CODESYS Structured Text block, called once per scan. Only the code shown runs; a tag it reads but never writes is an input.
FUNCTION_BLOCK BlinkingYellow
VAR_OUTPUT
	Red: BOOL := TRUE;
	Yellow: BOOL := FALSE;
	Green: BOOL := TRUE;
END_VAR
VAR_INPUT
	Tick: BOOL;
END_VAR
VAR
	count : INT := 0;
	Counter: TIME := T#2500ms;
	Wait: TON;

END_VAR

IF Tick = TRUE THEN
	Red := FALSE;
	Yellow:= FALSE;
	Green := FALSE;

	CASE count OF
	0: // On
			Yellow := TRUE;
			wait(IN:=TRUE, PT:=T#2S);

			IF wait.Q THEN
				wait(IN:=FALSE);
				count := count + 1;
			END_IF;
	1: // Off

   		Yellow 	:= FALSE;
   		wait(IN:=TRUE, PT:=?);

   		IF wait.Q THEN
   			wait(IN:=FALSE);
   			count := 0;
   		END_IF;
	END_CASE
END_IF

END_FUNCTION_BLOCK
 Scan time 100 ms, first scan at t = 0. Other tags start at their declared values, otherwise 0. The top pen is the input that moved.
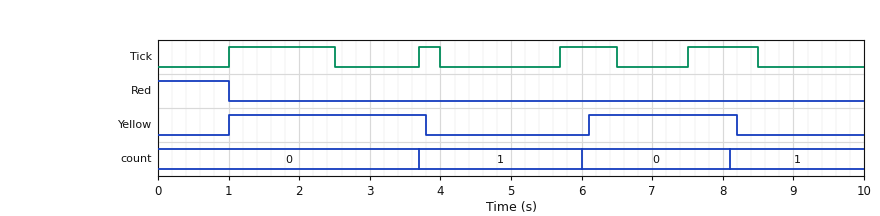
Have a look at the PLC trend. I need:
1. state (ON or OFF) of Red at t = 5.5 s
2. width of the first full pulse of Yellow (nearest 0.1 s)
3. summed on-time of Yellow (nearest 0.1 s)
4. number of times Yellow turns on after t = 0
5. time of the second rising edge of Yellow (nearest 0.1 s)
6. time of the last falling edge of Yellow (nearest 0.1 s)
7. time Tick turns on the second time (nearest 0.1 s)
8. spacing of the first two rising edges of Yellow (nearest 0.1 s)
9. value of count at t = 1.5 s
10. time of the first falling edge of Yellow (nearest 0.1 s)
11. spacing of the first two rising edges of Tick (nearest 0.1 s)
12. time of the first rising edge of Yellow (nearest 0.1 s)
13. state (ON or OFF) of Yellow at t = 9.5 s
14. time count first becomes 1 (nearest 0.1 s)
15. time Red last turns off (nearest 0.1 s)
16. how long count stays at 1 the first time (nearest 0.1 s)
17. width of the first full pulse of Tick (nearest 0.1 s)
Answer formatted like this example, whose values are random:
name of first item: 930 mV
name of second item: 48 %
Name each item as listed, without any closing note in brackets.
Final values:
state (ON or OFF) of Red at t = 5.5 s: OFF
width of the first full pulse of Yellow: 2.8 s
summed on-time of Yellow: 4.9 s
number of times Yellow turns on after t = 0: 2
time of the second rising edge of Yellow: 6.1 s
time of the last falling edge of Yellow: 8.2 s
time Tick turns on the second time: 3.7 s
spacing of the first two rising edges of Yellow: 5.1 s
value of count at t = 1.5 s: 0
time of the first falling edge of Yellow: 3.8 s
spacing of the first two rising edges of Tick: 2.7 s
time of the first rising edge of Yellow: 1.0 s
state (ON or OFF) of Yellow at t = 9.5 s: OFF
time count first becomes 1: 3.7 s
time Red last turns off: 1.0 s
how long count stays at 1 the first time: 2.3 s
width of the first full pulse of Tick: 1.5 s
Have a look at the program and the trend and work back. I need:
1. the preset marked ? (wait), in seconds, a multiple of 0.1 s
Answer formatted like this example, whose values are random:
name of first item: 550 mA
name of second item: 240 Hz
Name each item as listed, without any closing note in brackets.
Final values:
the preset marked ? (wait), in seconds, a multiple of 0.1 s: 2.2 s
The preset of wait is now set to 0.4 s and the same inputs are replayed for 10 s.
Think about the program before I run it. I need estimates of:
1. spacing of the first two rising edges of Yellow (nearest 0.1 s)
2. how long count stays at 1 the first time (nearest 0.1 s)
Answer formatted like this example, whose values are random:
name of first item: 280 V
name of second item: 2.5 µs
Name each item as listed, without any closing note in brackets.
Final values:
spacing of the first two rising edges of Yellow: 4.8 s
how long count stays at 1 the first time: 2.0 s
